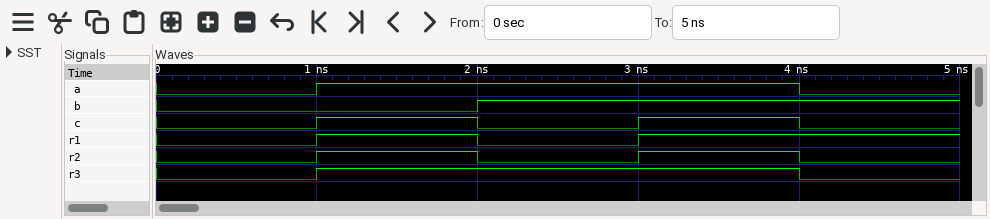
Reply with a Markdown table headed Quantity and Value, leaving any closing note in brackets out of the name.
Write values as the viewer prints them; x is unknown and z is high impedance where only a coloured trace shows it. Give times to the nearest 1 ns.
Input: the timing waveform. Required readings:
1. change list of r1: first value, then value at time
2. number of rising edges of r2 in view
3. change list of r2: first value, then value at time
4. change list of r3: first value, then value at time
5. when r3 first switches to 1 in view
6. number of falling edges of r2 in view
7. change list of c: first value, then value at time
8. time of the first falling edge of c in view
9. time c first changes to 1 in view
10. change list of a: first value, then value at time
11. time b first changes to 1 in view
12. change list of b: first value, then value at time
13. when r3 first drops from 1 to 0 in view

| Quantity | Value |
|---|---|
| change list of r1: first value, then value at time | 0, 1 at 1 ns, 0 at 2 ns, 1 at 3 ns |
| number of rising edges of r2 in view | 2 |
| change list of r2: first value, then value at time | 0, 1 at 1 ns, 0 at 2 ns, 1 at 3 ns, 0 at 4 ns |
| change list of r3: first value, then value at time | 0, 1 at 1 ns, 0 at 4 ns |
| when r3 first switches to 1 in view | 1 ns |
| number of falling edges of r2 in view | 2 |
| change list of c: first value, then value at time | 0, 1 at 1 ns, 0 at 2 ns, 1 at 3 ns, 0 at 4 ns |
| time of the first falling edge of c in view | 2 ns |
| time c first changes to 1 in view | 1 ns |
| change list of a: first value, then value at time | 0, 1 at 1 ns, 0 at 4 ns |
| time b first changes to 1 in view | 2 ns |
| change list of b: first value, then value at time | 0, 1 at 2 ns |
| when r3 first drops from 1 to 0 in view | 4 ns |
